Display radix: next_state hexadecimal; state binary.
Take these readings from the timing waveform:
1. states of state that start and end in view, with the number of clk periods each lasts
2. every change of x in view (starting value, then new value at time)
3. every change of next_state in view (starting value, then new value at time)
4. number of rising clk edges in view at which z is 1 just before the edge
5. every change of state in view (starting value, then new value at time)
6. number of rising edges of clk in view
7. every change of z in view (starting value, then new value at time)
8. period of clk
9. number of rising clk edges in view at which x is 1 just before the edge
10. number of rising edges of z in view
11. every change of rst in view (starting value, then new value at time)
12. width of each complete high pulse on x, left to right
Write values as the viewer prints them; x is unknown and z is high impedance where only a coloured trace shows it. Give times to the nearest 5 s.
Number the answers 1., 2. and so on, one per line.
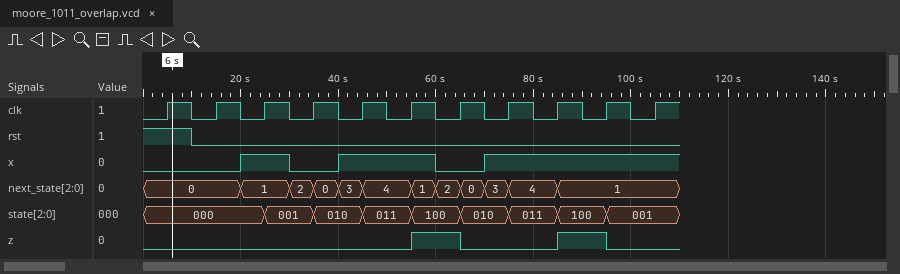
1. 001: 1, 010: 1, 011: 1, 100: 1, 010: 1, 011: 1, 100: 1
2. 0, 1 at 20 s, 0 at 30 s, 1 at 40 s, 0 at 60 s, 1 at 70 s
3. 0, 1 at 20 s, 2 at 30 s, 0 at 35 s, 3 at 40 s, 4 at 45 s, 1 at 55 s, 2 at 60 s, 0 at 65 s, 3 at 70 s, 4 at 75 s, 1 at 85 s
4. 2
5. 000, 001 at 25 s, 010 at 35 s, 011 at 45 s, 100 at 55 s, 010 at 65 s, 011 at 75 s, 100 at 85 s, 001 at 95 s
6. 11
7. 0, 1 at 55 s, 0 at 65 s, 1 at 85 s, 0 at 95 s
8. 10 s
9. 7
10. 2
11. 1, 0 at 10 s
12. 10 s, 20 s
